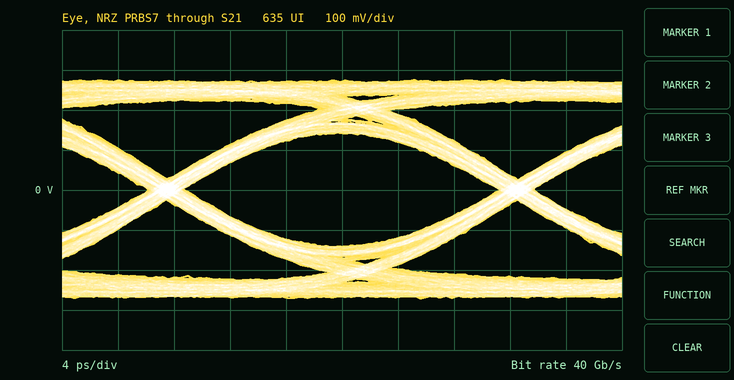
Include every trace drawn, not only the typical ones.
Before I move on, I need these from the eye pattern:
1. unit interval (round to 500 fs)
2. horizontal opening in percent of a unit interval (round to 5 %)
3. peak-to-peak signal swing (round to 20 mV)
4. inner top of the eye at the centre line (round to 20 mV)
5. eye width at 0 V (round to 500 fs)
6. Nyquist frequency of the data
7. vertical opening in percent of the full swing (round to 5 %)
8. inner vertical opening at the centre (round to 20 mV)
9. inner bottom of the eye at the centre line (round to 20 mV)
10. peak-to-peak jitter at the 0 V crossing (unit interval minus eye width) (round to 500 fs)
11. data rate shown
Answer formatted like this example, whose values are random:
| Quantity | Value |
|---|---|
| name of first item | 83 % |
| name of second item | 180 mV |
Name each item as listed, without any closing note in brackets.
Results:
| Quantity | Value |
|---|---|
| unit interval | 25.0 ps |
| horizontal opening in percent of a unit interval | 90 % |
| peak-to-peak signal swing | 540 mV |
| inner top of the eye at the centre line | 140 mV |
| eye width at 0 V | 22.5 ps |
| Nyquist frequency of the data | 20 GHz |
| vertical opening in percent of the full swing | 50 % |
| inner vertical opening at the centre | 280 mV |
| inner bottom of the eye at the centre line | -140 mV |
| peak-to-peak jitter at the 0 V crossing (unit interval minus eye width) | 2.5 ps |
| data rate shown | 40 Gb/s |
